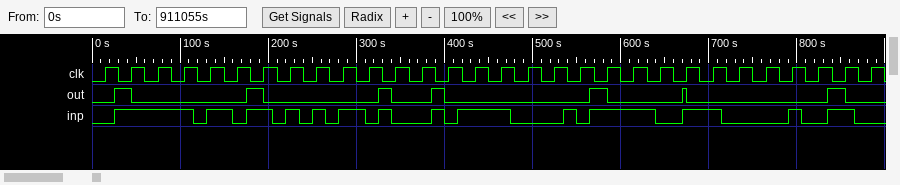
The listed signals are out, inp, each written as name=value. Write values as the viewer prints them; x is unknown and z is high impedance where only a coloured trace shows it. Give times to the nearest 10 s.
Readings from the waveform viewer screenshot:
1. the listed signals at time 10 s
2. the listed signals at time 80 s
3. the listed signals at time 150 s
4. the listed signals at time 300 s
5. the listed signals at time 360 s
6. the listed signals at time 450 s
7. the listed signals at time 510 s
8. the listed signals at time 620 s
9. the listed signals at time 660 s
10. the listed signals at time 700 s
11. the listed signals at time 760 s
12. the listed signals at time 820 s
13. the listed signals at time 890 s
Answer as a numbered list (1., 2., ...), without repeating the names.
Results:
1. out=0, inp=0
2. out=0, inp=1
3. out=0, inp=1
4. out=0, inp=1
5. out=0, inp=0
6. out=0, inp=1
7. out=0, inp=0
8. out=0, inp=1
9. out=0, inp=0
10. out=0, inp=1
11. out=0, inp=0
12. out=0, inp=0
13. out=0, inp=0
